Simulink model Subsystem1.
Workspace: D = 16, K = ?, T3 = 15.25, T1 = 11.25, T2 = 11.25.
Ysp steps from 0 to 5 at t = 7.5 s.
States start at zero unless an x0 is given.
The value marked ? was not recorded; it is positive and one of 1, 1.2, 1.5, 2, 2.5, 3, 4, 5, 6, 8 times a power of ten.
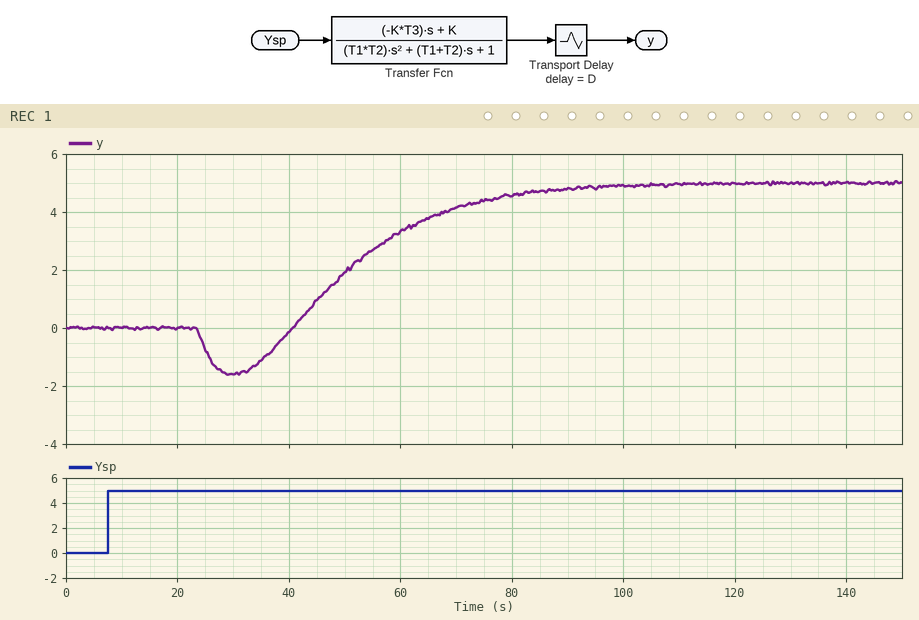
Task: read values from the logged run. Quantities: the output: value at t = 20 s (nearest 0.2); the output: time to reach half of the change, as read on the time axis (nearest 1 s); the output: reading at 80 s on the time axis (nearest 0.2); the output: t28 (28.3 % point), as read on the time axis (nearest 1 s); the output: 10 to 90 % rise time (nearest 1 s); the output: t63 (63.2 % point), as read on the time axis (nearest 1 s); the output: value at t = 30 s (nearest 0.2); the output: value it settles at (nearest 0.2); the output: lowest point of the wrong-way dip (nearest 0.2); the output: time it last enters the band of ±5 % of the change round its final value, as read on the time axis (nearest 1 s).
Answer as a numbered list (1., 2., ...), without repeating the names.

1. 0.0
2. 54 s
3. 4.6
4. 47 s
5. 35 s
6. 59 s
7. -1.6
8. 5.0
9. -1.6
10. 87 s
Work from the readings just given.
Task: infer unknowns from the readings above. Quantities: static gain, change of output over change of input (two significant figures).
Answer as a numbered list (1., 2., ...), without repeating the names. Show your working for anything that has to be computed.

1. (5 - 0) / (5 - 0) = 1.0
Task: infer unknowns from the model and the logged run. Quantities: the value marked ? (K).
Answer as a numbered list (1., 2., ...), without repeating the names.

1. 1
